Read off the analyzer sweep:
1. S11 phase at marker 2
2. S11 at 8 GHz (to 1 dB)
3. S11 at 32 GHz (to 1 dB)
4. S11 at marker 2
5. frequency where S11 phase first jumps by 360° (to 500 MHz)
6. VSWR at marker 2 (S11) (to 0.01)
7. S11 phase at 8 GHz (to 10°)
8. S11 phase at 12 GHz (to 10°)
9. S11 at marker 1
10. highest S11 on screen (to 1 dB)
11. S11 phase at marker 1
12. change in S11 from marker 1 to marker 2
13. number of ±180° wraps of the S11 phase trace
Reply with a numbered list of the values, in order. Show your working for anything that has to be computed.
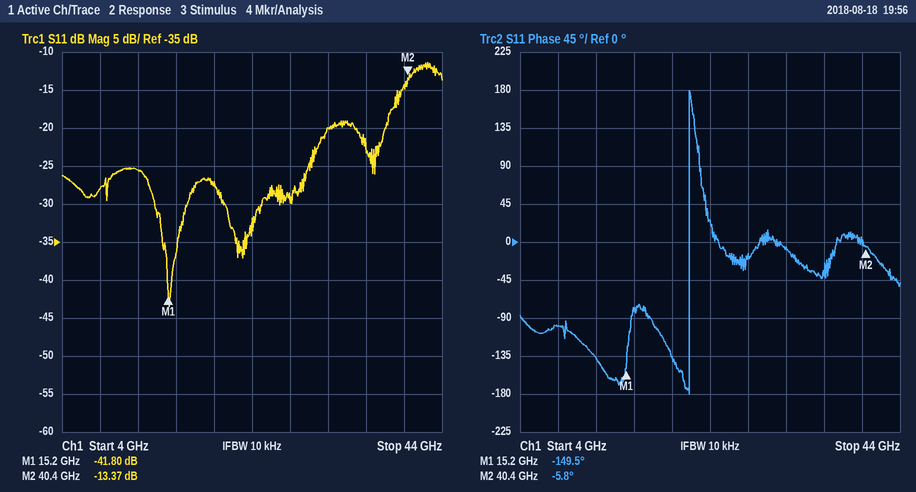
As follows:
1. -5.8°
2. -28 dB
3. -20 dB
4. -13.37 dB
5. 22.0 GHz
6. (1 + 0.2145)/(1 − 0.2145) ≈ 1.55
7. -100°
8. -140°
9. -41.80 dB
10. -11 dB
11. -149.5°
12. -13.37 − (-41.8) = 28.43 dB
13. 1
